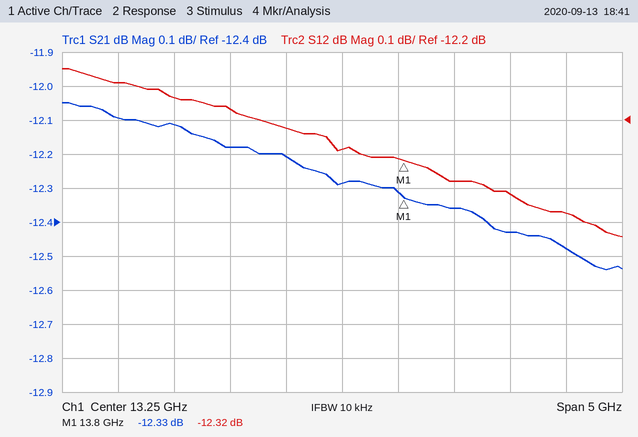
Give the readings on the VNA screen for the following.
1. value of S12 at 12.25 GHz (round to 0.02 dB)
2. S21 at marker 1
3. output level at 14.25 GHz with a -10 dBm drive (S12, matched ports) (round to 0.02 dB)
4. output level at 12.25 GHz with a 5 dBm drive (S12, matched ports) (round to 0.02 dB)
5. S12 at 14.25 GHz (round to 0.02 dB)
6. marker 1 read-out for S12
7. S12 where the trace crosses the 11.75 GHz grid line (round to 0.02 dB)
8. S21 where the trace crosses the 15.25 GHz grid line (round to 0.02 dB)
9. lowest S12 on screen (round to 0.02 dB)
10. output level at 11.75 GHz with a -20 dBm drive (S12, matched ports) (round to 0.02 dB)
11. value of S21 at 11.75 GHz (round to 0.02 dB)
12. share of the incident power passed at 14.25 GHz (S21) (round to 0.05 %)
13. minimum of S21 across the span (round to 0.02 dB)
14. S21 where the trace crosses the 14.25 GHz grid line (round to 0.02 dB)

-12.16 dB
-12.33 dB
-22.38 dBm
-7.16 dBm
-12.38 dB
-12.32 dB
-12.14 dB
-12.48 dB
-12.54 dB
-32.14 dBm
-12.12 dB
5.80 %
-12.54 dB
-12.36 dB
